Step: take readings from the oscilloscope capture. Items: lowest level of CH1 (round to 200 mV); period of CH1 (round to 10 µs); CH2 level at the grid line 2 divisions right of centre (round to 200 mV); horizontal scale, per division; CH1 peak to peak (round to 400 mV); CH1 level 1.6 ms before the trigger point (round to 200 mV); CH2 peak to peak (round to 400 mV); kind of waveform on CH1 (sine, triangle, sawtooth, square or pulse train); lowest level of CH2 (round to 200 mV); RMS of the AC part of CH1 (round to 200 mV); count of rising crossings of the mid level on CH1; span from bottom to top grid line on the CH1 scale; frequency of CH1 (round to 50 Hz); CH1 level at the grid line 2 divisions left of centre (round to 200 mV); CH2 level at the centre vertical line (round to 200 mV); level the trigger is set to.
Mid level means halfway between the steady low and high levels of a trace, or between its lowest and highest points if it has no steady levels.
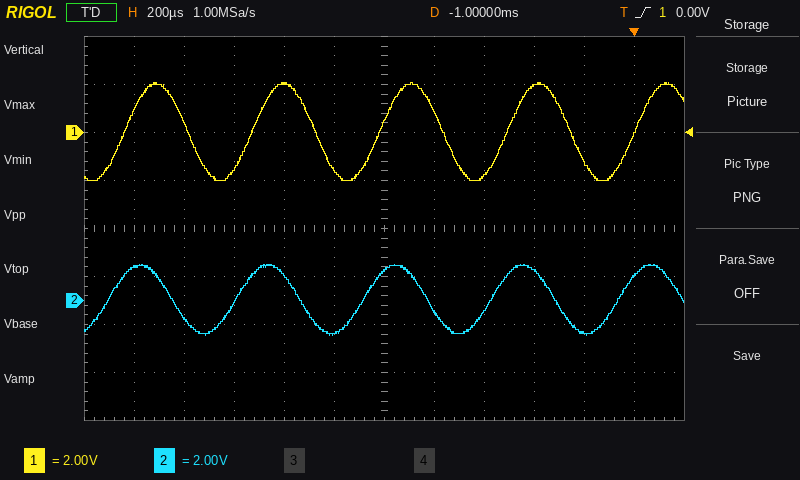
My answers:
-2.0 V
510 µs
-400 mV
200 µs
4.0 V
-1.6 V
2.8 V
sine
-1.4 V
1.4 V
5
16 V
1.95 kHz
2.0 V
1.2 V
0.00 V
